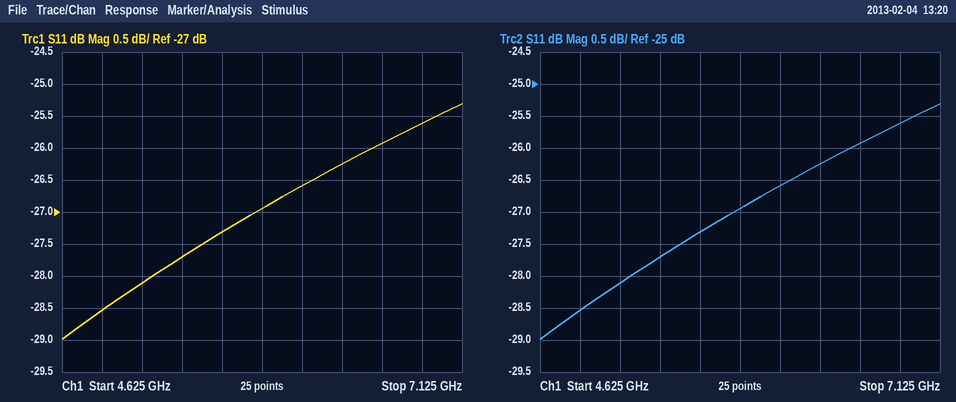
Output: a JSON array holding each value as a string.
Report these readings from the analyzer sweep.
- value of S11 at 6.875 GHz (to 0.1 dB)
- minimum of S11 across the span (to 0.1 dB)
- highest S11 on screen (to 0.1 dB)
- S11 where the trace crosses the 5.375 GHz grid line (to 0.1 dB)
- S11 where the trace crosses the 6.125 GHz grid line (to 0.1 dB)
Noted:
["-25.6 dB", "-29.0 dB", "-25.3 dB", "-27.7 dB", "-26.6 dB"]
